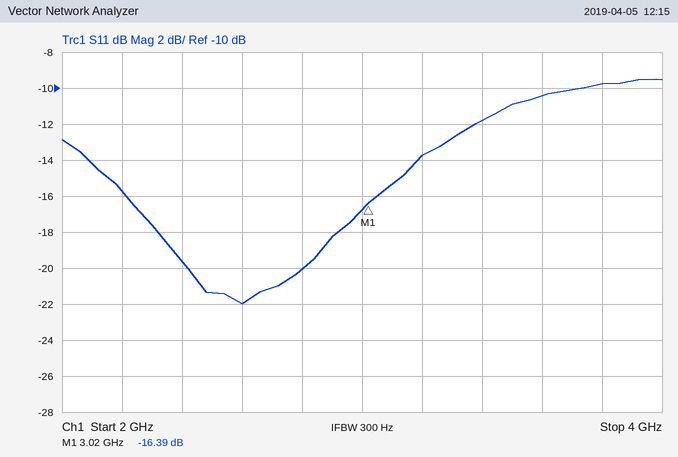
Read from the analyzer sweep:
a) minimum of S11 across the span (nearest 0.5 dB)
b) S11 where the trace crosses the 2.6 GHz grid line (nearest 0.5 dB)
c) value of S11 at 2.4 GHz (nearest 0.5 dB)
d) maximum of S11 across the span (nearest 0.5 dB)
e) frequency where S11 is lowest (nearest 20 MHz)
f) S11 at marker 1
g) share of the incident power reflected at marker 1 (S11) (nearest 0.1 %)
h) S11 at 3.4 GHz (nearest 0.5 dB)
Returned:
-22.0 dB
-22.0 dB
-19.5 dB
-9.5 dB
2.60 GHz
-16.39 dB
2.3 %
-12.0 dB
